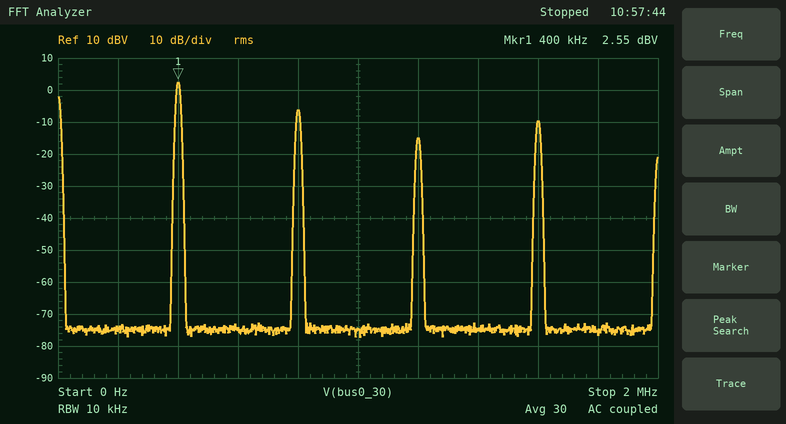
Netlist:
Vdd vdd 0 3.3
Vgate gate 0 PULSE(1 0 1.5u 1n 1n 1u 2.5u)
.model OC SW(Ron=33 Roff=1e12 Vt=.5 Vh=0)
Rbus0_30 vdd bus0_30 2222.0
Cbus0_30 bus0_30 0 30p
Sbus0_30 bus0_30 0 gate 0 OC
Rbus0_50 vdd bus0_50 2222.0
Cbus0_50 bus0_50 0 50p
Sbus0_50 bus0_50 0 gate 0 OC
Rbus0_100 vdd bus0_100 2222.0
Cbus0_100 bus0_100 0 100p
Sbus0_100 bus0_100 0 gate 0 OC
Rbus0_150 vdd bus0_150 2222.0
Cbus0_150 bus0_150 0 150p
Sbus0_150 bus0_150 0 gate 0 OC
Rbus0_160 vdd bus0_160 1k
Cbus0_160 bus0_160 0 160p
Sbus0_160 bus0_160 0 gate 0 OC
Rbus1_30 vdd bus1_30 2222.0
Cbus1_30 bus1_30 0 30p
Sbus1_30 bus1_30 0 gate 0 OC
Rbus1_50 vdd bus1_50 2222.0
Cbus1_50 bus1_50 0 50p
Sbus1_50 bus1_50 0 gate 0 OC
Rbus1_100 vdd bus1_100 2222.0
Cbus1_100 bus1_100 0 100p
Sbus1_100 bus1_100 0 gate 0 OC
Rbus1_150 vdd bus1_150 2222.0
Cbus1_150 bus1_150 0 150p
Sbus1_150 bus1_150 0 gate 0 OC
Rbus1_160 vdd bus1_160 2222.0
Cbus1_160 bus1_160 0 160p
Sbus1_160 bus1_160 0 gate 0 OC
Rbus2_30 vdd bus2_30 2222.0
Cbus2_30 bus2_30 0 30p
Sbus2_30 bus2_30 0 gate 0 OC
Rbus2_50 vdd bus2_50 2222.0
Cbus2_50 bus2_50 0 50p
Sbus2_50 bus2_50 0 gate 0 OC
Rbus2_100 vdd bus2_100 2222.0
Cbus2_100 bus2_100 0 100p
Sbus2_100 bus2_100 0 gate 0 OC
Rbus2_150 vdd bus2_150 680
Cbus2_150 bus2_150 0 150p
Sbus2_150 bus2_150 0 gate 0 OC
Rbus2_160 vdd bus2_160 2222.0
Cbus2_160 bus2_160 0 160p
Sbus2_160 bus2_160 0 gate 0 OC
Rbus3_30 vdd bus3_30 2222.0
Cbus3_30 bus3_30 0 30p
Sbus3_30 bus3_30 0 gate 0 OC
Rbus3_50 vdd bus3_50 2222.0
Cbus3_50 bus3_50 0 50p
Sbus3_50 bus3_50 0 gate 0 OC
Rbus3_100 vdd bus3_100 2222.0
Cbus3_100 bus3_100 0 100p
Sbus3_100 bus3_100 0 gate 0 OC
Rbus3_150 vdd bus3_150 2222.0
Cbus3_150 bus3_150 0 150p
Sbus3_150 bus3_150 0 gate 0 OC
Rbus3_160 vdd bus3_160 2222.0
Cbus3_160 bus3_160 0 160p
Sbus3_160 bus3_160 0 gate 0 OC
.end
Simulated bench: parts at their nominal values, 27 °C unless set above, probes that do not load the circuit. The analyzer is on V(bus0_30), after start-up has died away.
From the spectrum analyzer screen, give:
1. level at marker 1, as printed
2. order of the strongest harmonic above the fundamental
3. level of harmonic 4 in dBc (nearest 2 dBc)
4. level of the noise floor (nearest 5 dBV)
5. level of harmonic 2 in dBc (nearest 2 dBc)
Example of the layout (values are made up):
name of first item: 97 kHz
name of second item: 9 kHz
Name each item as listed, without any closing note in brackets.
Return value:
level at marker 1, as printed: 2.55 dBV
order of the strongest harmonic above the fundamental: 2
level of harmonic 4 in dBc: -12 dBc
level of the noise floor: -75 dBV
level of harmonic 2 in dBc: -8 dBc
